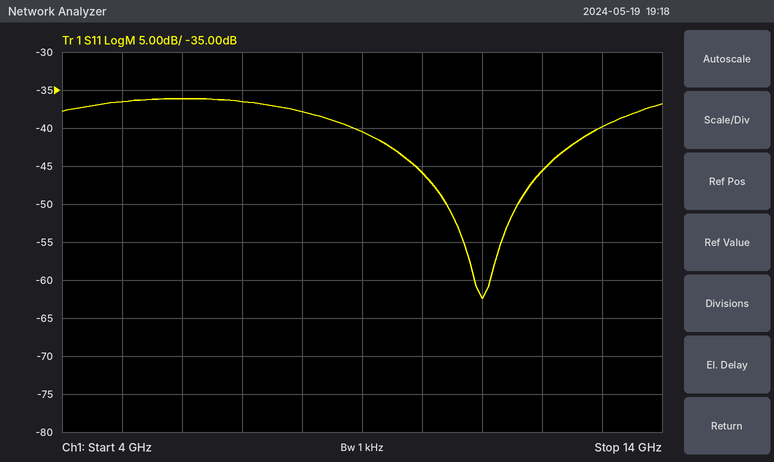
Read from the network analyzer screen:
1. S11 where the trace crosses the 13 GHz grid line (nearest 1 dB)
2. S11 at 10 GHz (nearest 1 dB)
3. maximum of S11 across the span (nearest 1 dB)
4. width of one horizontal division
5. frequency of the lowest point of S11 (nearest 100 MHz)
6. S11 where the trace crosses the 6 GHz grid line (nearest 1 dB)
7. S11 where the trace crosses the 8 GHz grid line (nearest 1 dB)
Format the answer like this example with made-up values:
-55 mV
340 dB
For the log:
-40 dB
-46 dB
-36 dB
1 GHz
11.0 GHz
-36 dB
-38 dB
